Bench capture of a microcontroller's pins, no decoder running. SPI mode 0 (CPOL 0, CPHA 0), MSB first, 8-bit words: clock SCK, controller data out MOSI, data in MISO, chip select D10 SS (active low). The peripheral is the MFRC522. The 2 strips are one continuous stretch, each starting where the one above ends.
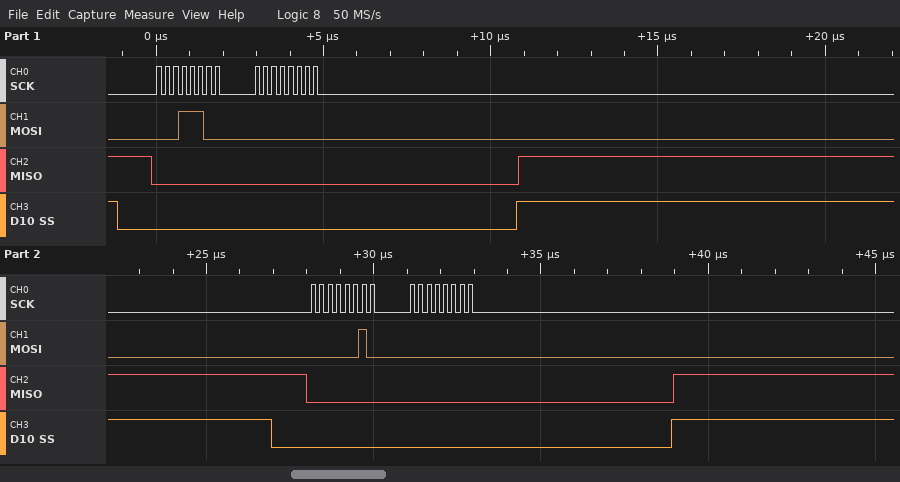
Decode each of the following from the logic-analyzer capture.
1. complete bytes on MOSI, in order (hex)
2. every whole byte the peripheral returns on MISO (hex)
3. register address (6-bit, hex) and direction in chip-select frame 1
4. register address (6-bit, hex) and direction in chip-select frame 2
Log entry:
1C 00 02 00
00 00 00 00
0x0E write
0x01 write
